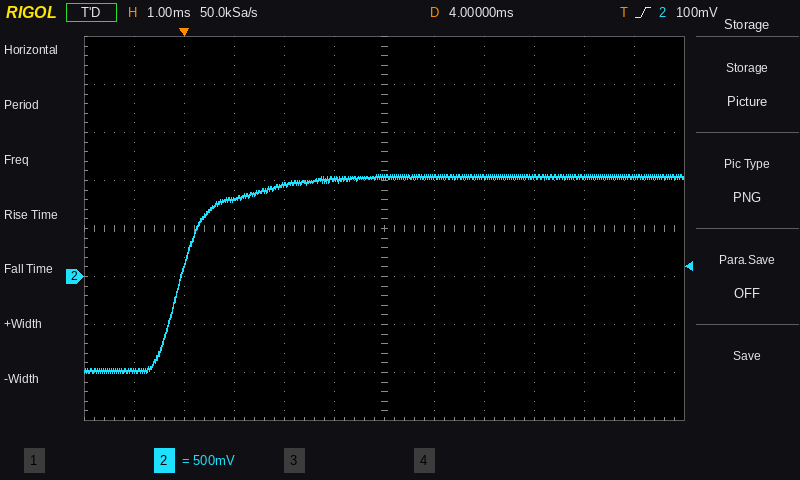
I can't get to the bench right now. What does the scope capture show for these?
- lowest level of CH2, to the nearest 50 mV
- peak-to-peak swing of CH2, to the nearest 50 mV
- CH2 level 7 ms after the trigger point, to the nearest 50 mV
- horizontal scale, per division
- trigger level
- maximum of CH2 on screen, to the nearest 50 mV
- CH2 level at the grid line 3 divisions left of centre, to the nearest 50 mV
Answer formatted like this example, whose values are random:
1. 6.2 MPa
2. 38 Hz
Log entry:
1. -1.00 V
2. 2.05 V
3. 1.05 V
4. 1 ms
5. 100 mV
6. 1.05 V
7. 800 mV
